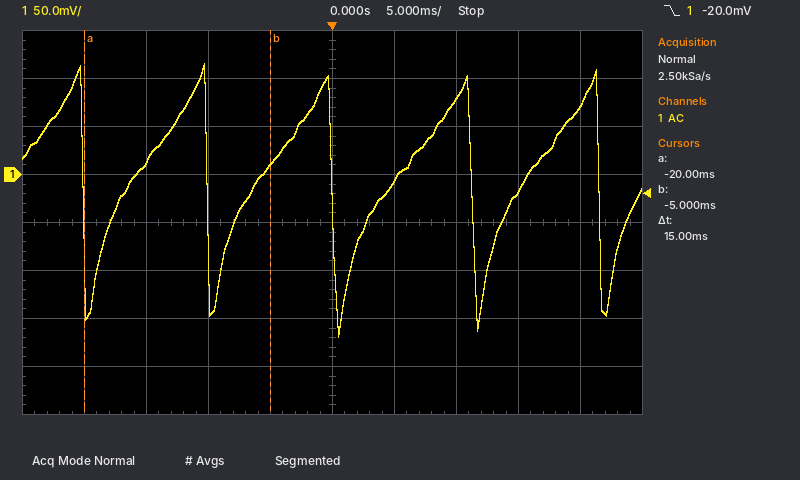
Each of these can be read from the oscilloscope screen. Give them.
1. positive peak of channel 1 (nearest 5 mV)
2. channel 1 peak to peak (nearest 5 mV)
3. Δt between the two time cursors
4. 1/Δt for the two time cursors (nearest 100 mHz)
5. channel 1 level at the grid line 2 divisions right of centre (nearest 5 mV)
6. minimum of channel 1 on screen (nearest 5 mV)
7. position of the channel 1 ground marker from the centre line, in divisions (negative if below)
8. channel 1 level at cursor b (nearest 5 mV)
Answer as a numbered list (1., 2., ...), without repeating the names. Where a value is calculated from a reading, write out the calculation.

1. 115 mV
2. 115 mV − (-170 mV) = 285 mV
3. 15 ms
4. 1 / 15 ms ≈ 66.7 Hz
5. 80 mV
6. -170 mV
7. +1.0 div
8. 10 mV
